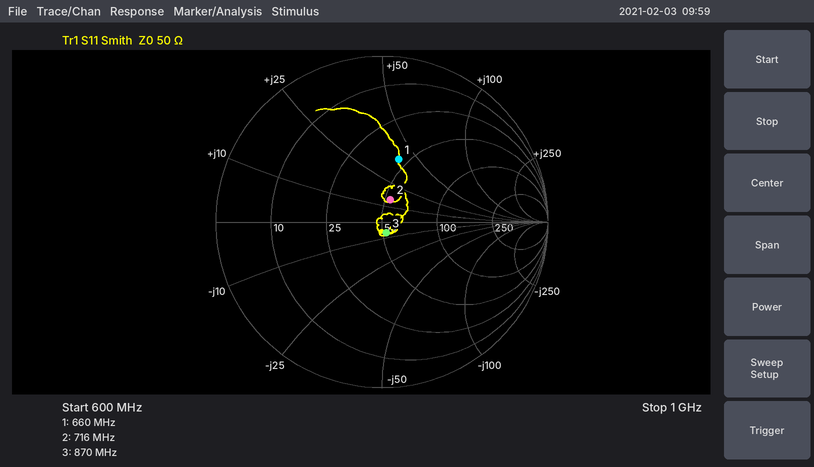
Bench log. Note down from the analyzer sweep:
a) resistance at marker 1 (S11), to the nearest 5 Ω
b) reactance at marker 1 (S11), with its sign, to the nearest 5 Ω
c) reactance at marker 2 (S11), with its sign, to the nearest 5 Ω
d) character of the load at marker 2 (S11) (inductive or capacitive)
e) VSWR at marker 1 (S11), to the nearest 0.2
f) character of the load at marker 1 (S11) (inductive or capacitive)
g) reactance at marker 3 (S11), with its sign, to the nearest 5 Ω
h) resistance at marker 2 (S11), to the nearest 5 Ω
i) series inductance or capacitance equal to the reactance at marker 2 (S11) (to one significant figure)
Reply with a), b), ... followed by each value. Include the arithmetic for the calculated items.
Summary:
a) 45 Ω
b) +40 Ω
c) +15 Ω
d) inductive
e) 2.2
f) inductive
g) -5 Ω
h) 55 Ω
i) L = 15 Ω/(2π × 716 MHz) ≈ 3 nH
